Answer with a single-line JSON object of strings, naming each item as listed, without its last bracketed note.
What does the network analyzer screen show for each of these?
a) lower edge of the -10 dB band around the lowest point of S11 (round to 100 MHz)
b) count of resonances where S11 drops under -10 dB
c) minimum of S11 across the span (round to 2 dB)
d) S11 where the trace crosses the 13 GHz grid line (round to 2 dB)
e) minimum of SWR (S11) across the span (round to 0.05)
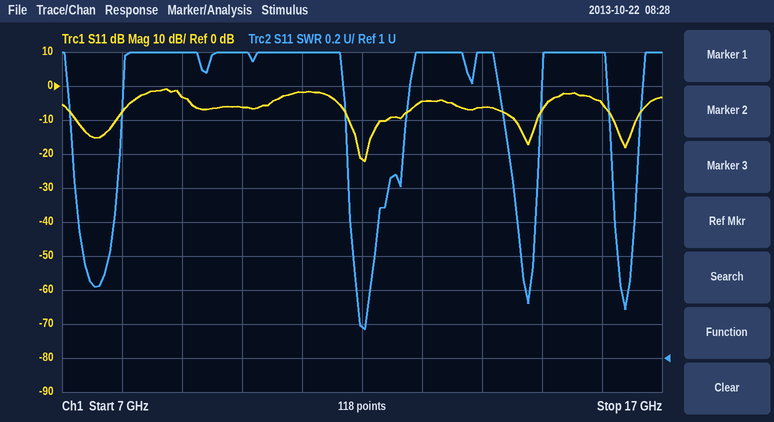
{"lower edge of the -10 dB band around the lowest point of S11": "11.8 GHz", "count of resonances where S11 drops under -10 dB": "4", "minimum of S11 across the span": "-22 dB", "S11 where the trace crosses the 13 GHz grid line": "-4 dB", "minimum of SWR (S11) across the span": "1.15"}
